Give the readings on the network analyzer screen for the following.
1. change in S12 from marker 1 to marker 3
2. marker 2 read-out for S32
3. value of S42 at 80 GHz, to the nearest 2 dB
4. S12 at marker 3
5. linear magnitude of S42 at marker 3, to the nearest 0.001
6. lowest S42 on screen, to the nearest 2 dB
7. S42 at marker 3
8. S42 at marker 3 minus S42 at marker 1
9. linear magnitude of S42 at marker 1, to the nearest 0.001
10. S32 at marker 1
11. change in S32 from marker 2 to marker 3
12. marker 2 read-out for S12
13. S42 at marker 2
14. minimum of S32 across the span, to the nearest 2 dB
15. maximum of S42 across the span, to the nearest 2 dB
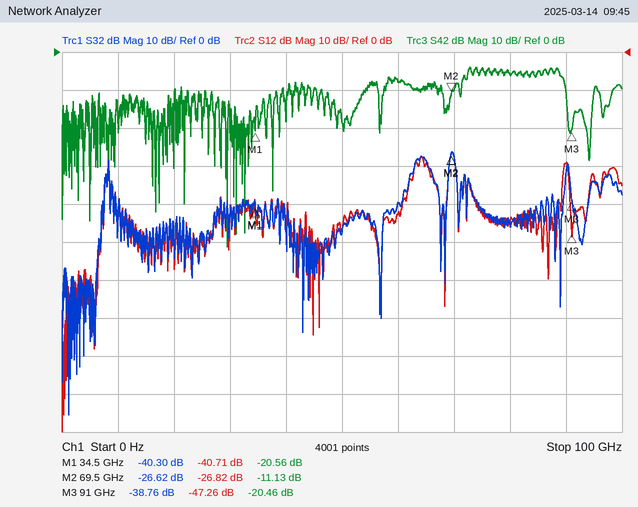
-6.55 dB
-26.62 dB
-6 dB
-47.26 dB
0.095
-52 dB
-20.46 dB
0.10 dB
0.094
-40.30 dB
-12.14 dB
-26.82 dB
-11.13 dB
-96 dB
-4 dB
